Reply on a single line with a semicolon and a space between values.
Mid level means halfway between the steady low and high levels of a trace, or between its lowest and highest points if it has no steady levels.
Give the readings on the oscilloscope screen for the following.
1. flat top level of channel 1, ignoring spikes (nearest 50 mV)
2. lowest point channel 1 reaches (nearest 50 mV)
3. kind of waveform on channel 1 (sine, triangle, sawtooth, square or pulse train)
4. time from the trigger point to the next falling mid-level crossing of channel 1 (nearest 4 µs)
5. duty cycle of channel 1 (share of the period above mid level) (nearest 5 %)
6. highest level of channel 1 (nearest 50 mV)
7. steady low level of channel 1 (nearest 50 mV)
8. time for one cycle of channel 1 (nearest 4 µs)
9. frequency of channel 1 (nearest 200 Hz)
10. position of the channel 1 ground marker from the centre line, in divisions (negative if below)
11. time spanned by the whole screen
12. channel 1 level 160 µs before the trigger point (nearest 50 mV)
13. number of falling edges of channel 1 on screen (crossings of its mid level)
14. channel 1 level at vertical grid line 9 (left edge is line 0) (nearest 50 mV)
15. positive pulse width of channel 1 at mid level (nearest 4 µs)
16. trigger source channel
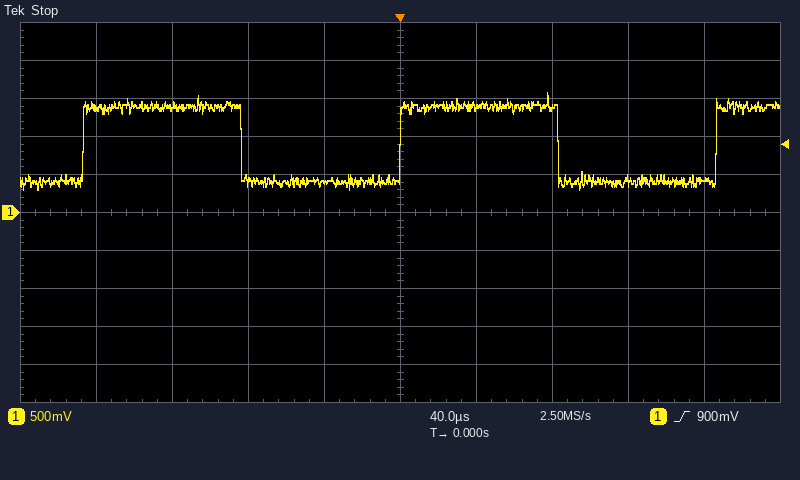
1.40 V; 300 mV; square; 84 µs; 50 %; 1.60 V; 400 mV; 168 µs; 6.0 kHz; 0.0 div; 400 µs; 1.40 V; 2; 450 mV; 84 µs; channel 1
